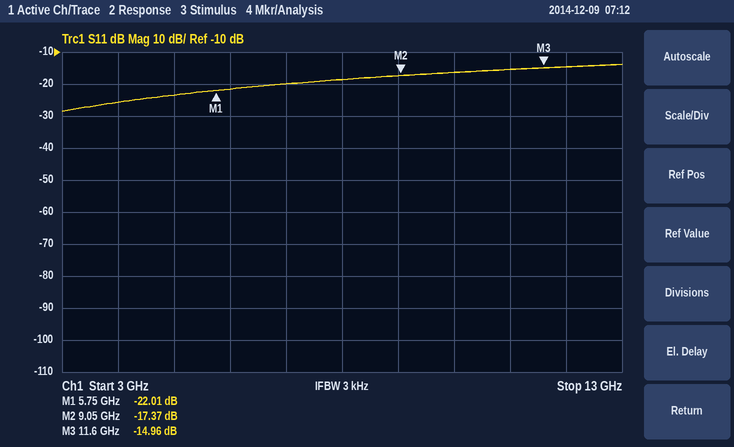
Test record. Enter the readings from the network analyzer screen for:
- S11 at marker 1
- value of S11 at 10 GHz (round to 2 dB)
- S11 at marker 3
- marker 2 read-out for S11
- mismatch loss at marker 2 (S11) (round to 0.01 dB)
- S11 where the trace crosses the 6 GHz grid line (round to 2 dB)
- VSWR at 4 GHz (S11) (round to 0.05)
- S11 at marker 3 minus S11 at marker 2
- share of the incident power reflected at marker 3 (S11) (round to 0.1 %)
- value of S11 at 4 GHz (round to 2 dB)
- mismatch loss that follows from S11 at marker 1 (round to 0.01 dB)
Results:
-22.01 dB
-16 dB
-14.96 dB
-17.37 dB
0.08 dB
-22 dB
1.10
2.41 dB
3.2 %
-26 dB
0.03 dB
